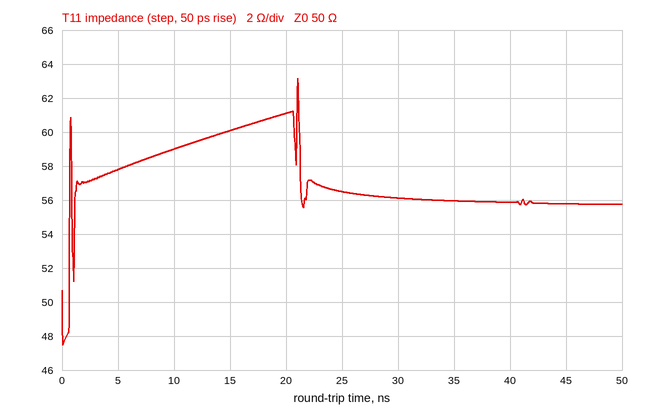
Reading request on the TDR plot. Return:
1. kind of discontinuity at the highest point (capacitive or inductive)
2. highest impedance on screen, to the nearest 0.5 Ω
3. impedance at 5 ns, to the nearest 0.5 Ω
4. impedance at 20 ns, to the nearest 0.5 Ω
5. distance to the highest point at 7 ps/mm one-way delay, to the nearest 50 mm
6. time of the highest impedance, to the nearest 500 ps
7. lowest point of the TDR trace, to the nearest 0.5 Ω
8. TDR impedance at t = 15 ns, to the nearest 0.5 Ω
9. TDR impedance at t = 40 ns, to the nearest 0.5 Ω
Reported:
inductive
63.0 Ω
58.0 Ω
61.0 Ω
1.50 m
21.0 ns
47.5 Ω
60.0 Ω
56.0 Ω
